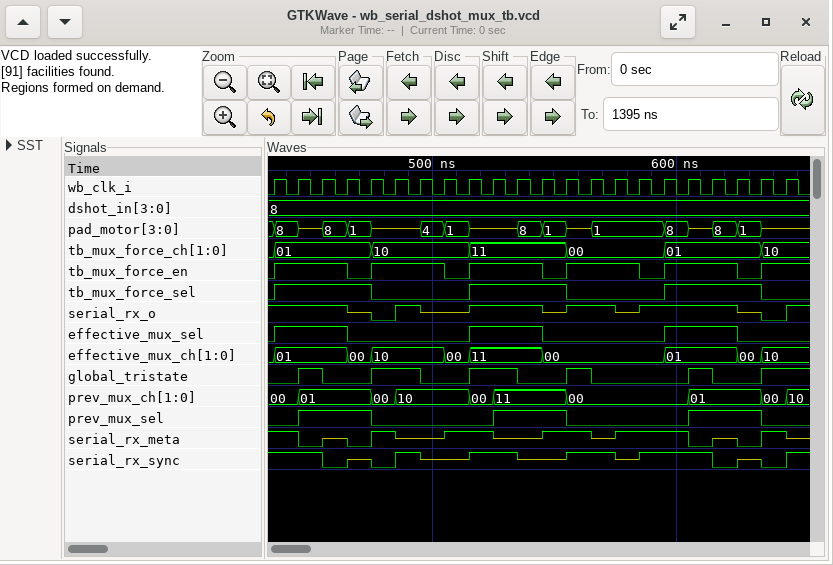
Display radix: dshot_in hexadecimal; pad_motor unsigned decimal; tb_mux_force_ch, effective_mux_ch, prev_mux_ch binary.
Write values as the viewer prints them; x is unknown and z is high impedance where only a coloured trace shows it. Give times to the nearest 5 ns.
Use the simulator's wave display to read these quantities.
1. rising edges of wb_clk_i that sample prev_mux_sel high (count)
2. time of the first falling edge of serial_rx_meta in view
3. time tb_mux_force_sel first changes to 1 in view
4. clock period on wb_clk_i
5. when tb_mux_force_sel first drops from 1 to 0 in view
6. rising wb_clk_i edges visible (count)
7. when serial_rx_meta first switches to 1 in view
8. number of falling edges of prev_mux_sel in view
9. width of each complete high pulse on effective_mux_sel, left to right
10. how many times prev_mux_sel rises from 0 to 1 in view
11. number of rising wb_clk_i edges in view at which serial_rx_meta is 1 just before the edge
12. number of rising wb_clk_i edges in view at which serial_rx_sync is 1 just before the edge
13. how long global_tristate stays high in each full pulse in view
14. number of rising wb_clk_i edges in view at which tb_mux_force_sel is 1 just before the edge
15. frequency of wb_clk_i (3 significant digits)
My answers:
9
445 ns
435 ns
10 ns
475 ns
22
475 ns
3
30 ns, 30 ns, 30 ns
3
11
11
10 ns, 20 ns, 20 ns, 10 ns, 10 ns
12
100 MHz
